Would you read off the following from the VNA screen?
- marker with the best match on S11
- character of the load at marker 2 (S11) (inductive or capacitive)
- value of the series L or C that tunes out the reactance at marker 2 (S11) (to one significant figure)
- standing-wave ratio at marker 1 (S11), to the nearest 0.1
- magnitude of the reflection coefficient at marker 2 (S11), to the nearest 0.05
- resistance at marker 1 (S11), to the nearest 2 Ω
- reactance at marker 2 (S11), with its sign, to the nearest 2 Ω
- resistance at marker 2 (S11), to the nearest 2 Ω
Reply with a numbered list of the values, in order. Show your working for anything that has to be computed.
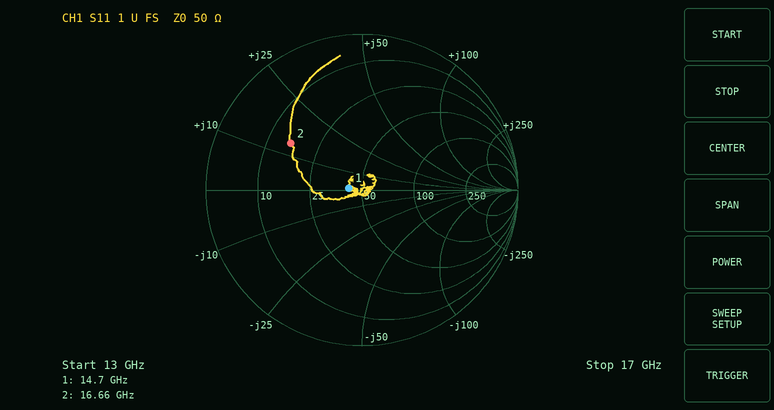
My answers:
1. marker 1
2. inductive
3. C = 1/(2π × 16.66 GHz × 14 Ω) ≈ 682 fF, so 700 fF to one significant figure
4. 1.2
5. 0.55
6. 42 Ω
7. +14 Ω
8. 16 Ω
